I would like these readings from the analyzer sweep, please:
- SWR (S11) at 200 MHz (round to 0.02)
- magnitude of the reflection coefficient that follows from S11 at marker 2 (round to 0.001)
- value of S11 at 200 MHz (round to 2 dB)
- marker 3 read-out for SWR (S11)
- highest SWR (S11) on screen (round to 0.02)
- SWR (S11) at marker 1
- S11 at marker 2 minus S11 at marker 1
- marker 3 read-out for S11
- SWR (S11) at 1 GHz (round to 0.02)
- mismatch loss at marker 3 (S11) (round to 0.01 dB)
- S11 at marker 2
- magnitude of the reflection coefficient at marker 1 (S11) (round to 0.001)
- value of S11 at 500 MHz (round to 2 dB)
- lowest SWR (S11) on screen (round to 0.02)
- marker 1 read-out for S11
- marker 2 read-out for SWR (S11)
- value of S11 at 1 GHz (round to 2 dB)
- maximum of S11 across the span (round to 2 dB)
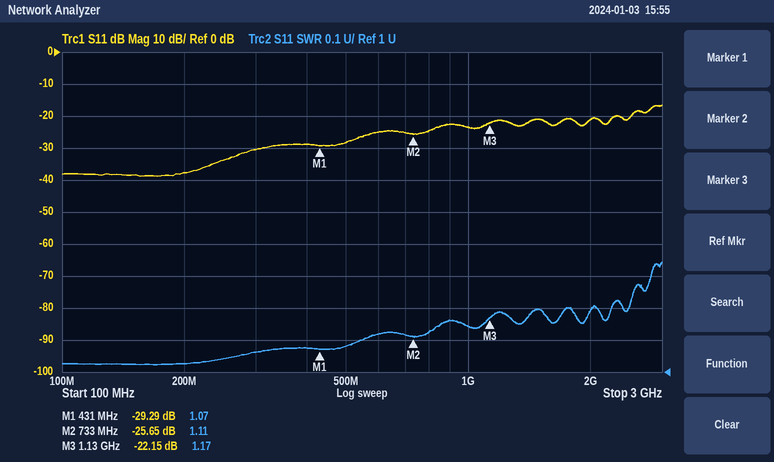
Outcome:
1.02
0.052
-38 dB
1.17
1.34
1.07
3.64 dB
-22.15 dB
1.14
0.03 dB
-25.65 dB
0.034
-28 dB
1.02
-29.29 dB
1.11
-24 dB
-16 dB
